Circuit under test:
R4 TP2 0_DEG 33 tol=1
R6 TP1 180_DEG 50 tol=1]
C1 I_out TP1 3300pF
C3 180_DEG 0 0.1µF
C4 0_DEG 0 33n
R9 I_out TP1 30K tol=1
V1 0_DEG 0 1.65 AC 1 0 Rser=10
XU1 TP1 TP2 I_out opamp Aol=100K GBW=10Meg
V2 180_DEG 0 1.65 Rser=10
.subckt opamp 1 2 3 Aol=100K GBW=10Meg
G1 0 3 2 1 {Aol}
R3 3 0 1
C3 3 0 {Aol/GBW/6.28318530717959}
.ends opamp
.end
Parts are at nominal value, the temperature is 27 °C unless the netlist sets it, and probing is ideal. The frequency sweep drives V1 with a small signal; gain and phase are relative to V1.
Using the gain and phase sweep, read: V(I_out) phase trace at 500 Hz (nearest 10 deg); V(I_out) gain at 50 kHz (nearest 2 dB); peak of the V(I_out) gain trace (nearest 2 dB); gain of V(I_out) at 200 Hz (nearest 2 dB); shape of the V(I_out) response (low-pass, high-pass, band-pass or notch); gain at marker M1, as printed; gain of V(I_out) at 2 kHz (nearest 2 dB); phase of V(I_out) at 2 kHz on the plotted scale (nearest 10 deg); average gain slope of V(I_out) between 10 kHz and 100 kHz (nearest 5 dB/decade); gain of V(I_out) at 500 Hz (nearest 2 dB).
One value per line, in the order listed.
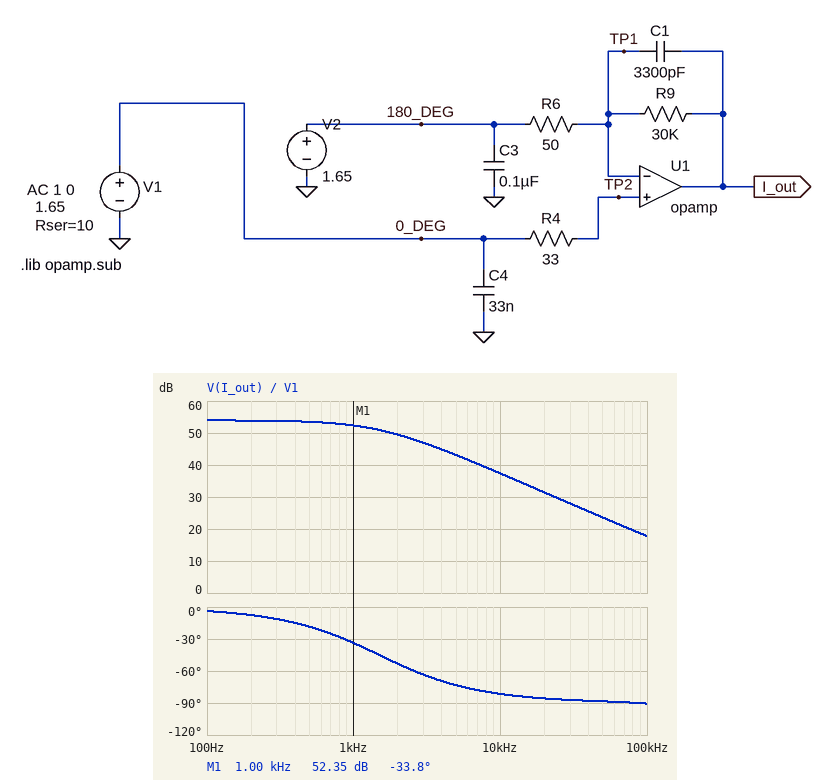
-20 deg
24 dB
54 dB
54 dB
low-pass
52.35 dB
50 dB
-50 deg
-20 dB/decade
54 dB
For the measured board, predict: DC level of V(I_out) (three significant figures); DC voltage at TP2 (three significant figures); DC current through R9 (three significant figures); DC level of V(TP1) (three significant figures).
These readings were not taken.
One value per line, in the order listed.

1.64 V
1.65 V
274 nA
1.65 V
